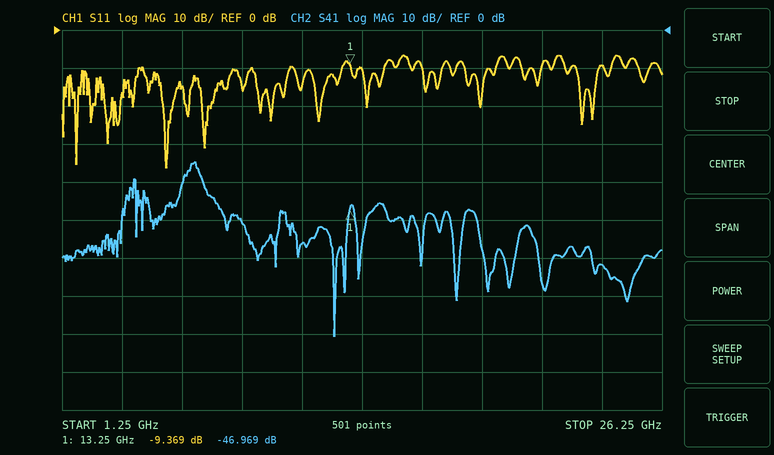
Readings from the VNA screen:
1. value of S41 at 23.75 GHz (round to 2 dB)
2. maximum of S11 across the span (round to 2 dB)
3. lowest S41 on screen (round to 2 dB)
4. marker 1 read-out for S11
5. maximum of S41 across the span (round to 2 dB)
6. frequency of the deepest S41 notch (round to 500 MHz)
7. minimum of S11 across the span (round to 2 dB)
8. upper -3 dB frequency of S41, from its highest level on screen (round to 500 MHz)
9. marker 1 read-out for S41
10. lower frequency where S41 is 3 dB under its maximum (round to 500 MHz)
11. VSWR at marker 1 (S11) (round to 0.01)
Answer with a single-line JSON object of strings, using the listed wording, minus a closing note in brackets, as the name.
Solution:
{"value of S41 at 23.75 GHz": "-62 dB", "maximum of S11 across the span": "-6 dB", "lowest S41 on screen": "-80 dB", "marker 1 read-out for S11": "-9.369 dB", "maximum of S41 across the span": "-34 dB", "frequency of the deepest S41 notch": "12.5 GHz", "minimum of S11 across the span": "-36 dB", "upper -3 dB frequency of S41, from its highest level on screen": "7.0 GHz", "marker 1 read-out for S41": "-46.969 dB", "lower frequency where S41 is 3 dB under its maximum": "6.5 GHz", "VSWR at marker 1 (S11)": "2.03"}
